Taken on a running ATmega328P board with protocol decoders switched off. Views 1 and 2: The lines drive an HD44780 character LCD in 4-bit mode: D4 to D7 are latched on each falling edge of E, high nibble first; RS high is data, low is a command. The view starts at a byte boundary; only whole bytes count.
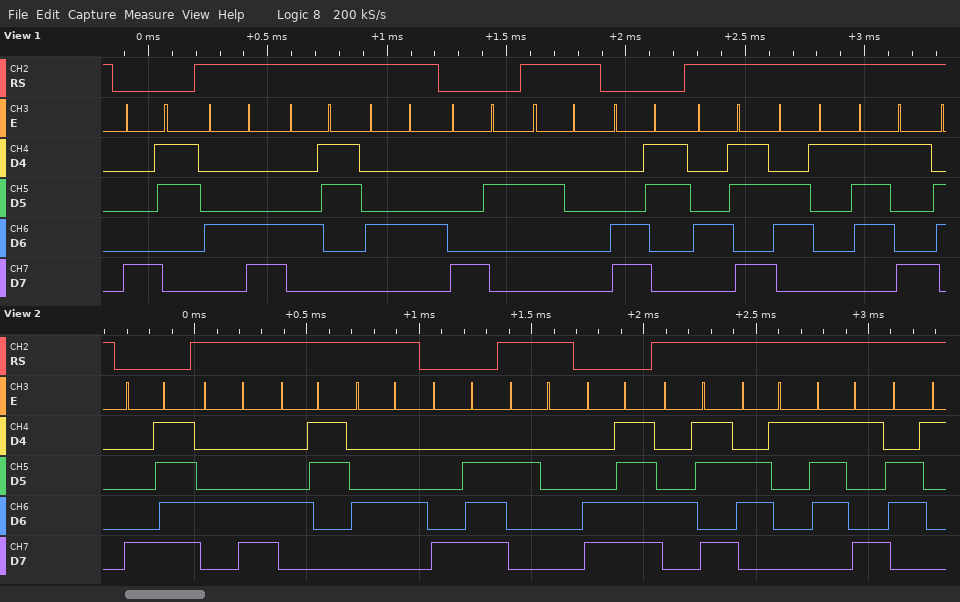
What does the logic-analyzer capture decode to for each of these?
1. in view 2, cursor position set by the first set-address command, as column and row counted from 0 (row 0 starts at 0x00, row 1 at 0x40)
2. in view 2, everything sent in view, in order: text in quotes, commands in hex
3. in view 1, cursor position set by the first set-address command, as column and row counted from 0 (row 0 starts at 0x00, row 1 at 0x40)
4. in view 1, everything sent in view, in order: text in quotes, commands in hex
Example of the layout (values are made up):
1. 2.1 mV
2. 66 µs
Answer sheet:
1. column 15, row 0
2. 0x8F "LCD" 0x8E " " 0xCF "Kaya"
3. column 3, row 0
4. 0x83 "LCD" 0x82 " " 0xC3 "Kay"
